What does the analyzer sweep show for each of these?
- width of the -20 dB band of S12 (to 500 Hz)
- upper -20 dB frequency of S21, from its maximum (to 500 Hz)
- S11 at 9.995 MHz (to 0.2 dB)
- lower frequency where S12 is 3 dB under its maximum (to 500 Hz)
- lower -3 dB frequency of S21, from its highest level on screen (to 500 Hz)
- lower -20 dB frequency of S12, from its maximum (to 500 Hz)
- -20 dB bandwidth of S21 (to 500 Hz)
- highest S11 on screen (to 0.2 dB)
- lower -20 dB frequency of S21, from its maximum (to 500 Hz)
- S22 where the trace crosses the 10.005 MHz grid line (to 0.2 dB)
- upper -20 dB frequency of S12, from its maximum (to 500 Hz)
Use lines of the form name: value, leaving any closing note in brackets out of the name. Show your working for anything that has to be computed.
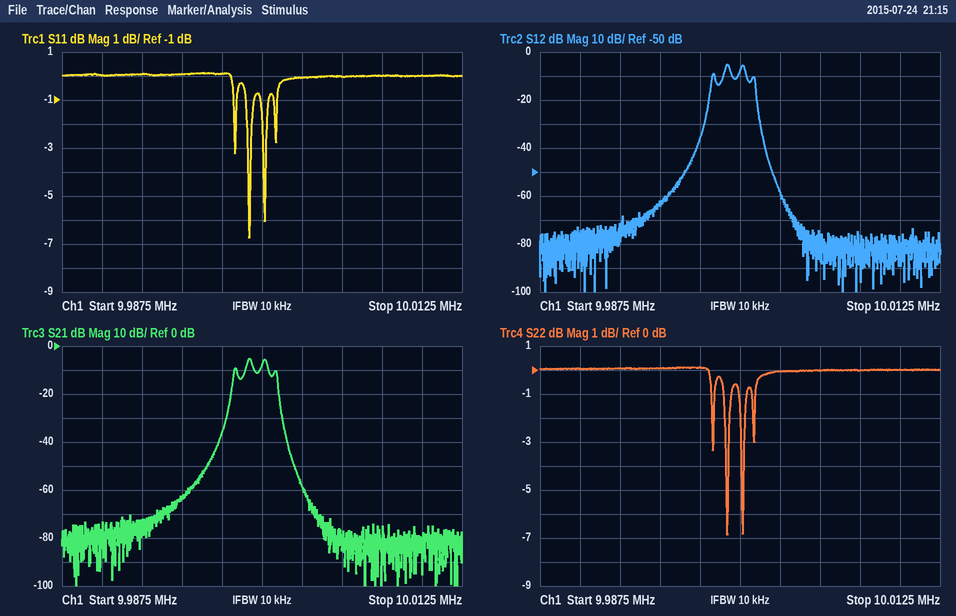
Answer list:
width of the -20 dB band of S12: 10.0010 MHz − 9.9980 MHz = 3.0 kHz
upper -20 dB frequency of S21, from its maximum: 10.0010 MHz
S11 at 9.995 MHz: 0.0 dB
lower frequency where S12 is 3 dB under its maximum: 9.9990 MHz
lower -3 dB frequency of S21, from its highest level on screen: 9.9990 MHz
lower -20 dB frequency of S12, from its maximum: 9.9980 MHz
-20 dB bandwidth of S21: 10.0010 MHz − 9.9980 MHz = 3.0 kHz
highest S11 on screen: 0.2 dB
lower -20 dB frequency of S21, from its maximum: 9.9980 MHz
S22 where the trace crosses the 10.005 MHz grid line: 0.0 dB
upper -20 dB frequency of S12, from its maximum: 10.0010 MHz
